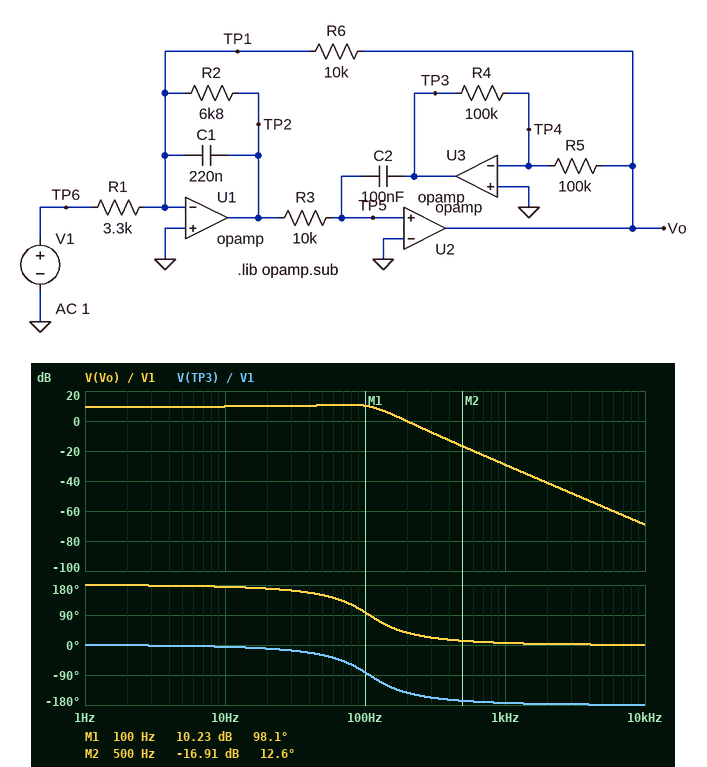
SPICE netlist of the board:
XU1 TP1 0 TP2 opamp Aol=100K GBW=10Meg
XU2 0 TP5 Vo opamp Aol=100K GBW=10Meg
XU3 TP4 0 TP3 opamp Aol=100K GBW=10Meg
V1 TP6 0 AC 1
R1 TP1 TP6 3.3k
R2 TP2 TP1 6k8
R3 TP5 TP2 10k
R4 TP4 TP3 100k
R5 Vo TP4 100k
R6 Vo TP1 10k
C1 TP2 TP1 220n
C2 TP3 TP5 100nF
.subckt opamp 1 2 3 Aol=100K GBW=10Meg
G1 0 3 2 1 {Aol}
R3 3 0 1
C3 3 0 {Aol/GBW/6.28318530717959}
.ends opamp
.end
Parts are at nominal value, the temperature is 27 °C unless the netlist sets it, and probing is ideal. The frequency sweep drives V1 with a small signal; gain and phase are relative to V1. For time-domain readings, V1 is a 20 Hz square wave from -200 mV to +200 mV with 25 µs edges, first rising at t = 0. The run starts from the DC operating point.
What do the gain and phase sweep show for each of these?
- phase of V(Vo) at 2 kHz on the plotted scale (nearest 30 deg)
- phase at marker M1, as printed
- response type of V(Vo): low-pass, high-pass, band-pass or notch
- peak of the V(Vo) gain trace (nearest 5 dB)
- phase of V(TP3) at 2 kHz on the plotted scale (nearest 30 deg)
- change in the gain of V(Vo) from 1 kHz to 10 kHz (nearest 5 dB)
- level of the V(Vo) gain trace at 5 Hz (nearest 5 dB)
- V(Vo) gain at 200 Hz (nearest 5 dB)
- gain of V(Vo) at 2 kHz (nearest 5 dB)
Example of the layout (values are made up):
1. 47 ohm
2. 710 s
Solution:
1. 0 deg
2. 98.1 deg
3. low-pass
4. 10 dB
5. -180 deg
6. -40 dB
7. 10 dB
8. 0 dB
9. -40 dB
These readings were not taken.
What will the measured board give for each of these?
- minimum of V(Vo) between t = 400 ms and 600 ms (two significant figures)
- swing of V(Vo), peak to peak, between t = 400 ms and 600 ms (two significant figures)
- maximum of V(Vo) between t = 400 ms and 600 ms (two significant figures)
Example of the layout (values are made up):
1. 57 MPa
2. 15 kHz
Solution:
1. -810 mV
2. 1.6 V
3. 810 mV
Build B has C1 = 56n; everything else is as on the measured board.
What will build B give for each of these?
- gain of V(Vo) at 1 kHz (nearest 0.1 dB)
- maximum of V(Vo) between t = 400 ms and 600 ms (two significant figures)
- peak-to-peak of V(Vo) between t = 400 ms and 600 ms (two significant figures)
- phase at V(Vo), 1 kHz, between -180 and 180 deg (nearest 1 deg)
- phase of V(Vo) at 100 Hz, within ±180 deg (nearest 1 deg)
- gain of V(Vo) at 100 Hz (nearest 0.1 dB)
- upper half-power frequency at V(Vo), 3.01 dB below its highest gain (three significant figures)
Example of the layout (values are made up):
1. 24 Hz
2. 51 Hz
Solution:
1. -17.6 dB
2. 610 mV
3. 1.2 V
4. 24 deg
5. 130 deg
6. 8.0 dB
7. 140 Hz
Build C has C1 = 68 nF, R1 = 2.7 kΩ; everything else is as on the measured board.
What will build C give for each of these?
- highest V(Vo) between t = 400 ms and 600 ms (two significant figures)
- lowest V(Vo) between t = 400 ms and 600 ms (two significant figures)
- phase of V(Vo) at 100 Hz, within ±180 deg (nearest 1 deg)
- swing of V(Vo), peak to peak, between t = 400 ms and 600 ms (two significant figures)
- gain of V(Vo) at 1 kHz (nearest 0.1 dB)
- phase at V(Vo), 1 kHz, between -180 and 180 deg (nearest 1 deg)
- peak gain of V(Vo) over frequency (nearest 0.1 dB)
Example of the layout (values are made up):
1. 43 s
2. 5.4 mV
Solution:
1. 740 mV
2. -740 mV
3. 128 deg
4. 1.5 V
5. -17.4 dB
6. 20 deg
7. 11.4 dB
